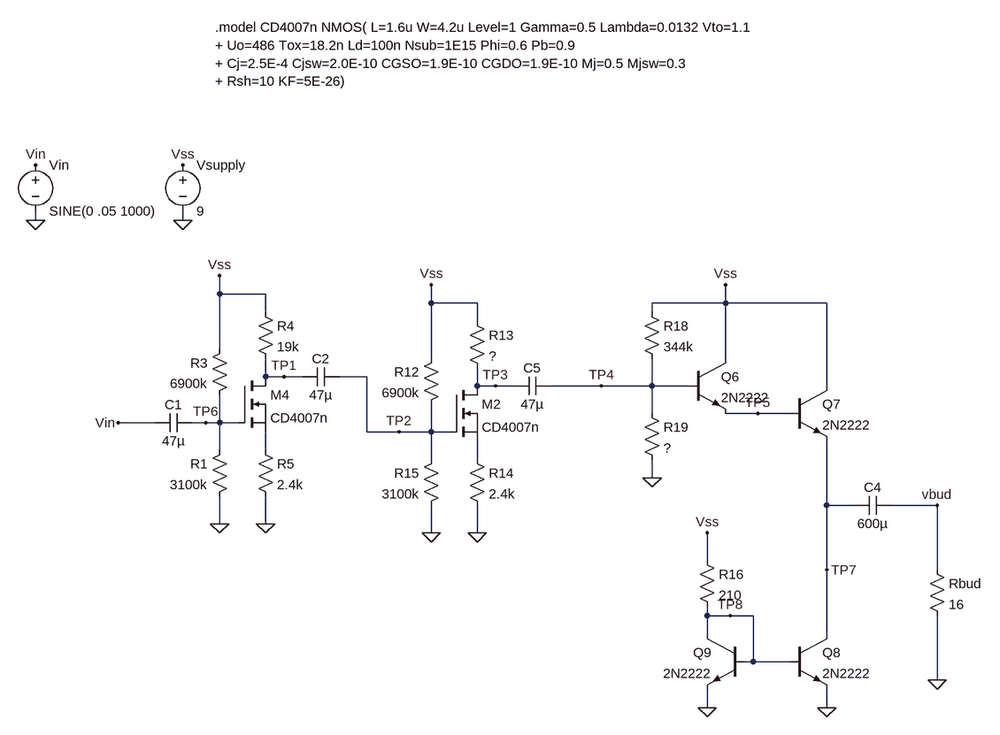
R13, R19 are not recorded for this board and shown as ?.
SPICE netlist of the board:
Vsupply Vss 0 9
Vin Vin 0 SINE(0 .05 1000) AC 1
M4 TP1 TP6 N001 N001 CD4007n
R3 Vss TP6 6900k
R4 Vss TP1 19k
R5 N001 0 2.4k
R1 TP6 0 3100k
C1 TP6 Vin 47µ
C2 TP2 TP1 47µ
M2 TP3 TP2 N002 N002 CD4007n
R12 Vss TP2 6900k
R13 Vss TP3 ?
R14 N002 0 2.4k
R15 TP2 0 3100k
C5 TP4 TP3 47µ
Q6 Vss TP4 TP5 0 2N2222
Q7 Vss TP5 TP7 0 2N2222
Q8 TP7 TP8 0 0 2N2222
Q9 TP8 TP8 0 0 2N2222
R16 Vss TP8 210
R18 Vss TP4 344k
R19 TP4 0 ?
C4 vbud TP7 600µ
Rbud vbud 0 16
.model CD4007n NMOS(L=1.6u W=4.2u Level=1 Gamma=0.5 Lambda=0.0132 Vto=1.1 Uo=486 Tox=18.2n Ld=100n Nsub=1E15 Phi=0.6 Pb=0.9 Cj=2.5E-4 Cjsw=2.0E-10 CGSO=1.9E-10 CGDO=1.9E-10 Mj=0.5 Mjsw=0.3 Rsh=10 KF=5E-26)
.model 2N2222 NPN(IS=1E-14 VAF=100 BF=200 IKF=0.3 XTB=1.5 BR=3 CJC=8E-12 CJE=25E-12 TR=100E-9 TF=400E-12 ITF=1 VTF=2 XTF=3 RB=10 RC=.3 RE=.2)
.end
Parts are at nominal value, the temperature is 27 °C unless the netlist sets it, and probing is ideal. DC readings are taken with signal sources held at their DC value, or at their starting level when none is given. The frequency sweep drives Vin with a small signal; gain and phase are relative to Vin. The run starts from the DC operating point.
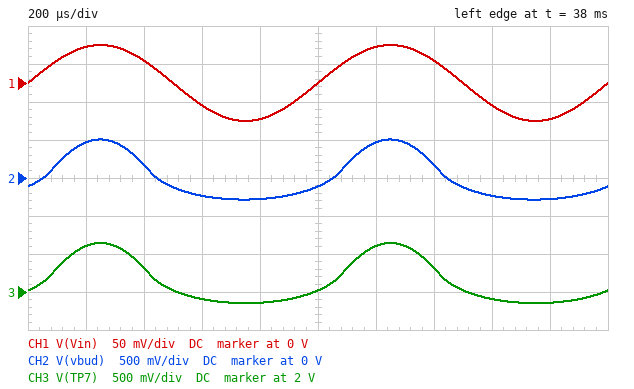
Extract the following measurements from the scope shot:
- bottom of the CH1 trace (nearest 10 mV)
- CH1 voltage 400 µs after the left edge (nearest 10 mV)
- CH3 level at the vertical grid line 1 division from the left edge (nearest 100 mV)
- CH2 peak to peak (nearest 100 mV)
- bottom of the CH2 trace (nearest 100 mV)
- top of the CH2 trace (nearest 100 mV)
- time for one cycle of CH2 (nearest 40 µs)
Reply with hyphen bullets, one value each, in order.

- -50 mV
- 30 mV
- 2.6 V
- 800 mV
- -300 mV
- 500 mV
- 1.00 ms
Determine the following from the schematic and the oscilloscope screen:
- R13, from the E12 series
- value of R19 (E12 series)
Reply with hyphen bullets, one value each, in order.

- 39 kΩ
- 220 kΩ
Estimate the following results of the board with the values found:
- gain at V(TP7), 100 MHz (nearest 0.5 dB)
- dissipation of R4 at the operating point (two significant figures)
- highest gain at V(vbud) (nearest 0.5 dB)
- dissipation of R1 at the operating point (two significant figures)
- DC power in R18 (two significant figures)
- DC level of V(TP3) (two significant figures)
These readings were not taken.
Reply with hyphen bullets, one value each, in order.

- -34.5 dB
- 820 µW
- 14.5 dB
- 2.5 µW
- 92 µW
- 1.4 V
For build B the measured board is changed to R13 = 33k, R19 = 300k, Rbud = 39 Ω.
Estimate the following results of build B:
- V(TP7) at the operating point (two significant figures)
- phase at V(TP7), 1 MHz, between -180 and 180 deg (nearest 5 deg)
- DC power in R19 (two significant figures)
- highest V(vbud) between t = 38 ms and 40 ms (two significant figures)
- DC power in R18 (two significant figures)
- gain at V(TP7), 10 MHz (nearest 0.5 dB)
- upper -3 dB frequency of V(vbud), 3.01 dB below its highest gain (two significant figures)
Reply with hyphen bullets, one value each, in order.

- 2.7 V
- -40 deg
- 54 µW
- 770 mV
- 72 µW
- 2.5 dB
- 1.4 MHz
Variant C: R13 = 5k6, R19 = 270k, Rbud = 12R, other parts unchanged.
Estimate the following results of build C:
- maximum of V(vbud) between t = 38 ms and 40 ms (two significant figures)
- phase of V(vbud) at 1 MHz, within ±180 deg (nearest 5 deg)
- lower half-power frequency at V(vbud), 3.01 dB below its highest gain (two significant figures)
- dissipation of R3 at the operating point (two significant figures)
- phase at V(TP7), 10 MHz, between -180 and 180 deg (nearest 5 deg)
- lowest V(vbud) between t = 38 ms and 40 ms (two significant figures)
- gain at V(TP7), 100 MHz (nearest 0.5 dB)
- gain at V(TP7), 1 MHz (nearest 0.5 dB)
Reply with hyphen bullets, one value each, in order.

- 150 mV
- -15 deg
- 20 Hz
- 5.6 µW
- -125 deg
- -150 mV
- -33.5 dB
- 10.0 dB
